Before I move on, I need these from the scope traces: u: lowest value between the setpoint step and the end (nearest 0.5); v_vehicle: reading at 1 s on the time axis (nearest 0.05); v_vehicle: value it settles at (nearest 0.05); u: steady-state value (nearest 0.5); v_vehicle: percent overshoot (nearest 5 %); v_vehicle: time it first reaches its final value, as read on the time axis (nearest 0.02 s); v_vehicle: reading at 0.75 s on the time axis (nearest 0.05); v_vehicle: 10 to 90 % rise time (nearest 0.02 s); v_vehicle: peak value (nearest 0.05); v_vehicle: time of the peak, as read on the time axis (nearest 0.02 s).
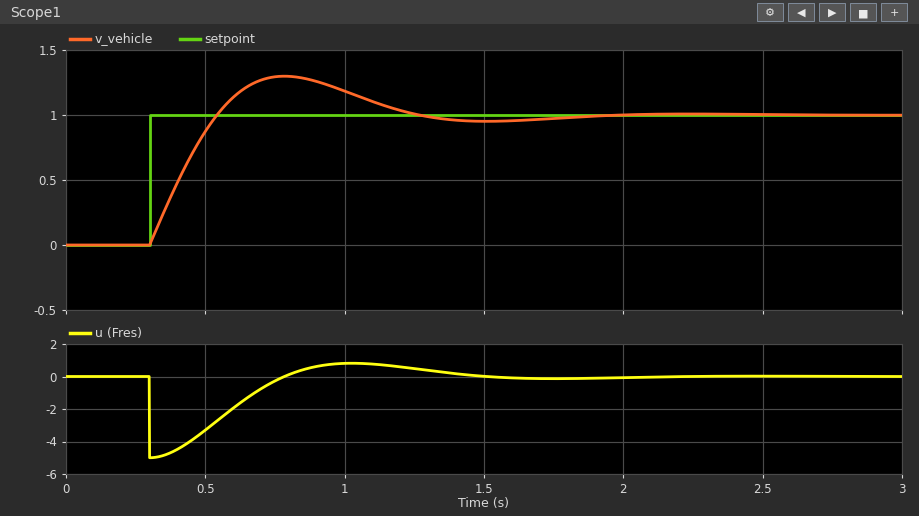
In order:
-5.0
1.20
1.00
0.0
30 %
0.54 s
1.30
0.18 s
1.30
0.78 s
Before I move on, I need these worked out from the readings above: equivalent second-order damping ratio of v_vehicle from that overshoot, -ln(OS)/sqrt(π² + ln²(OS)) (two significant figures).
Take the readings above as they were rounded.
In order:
0.36
